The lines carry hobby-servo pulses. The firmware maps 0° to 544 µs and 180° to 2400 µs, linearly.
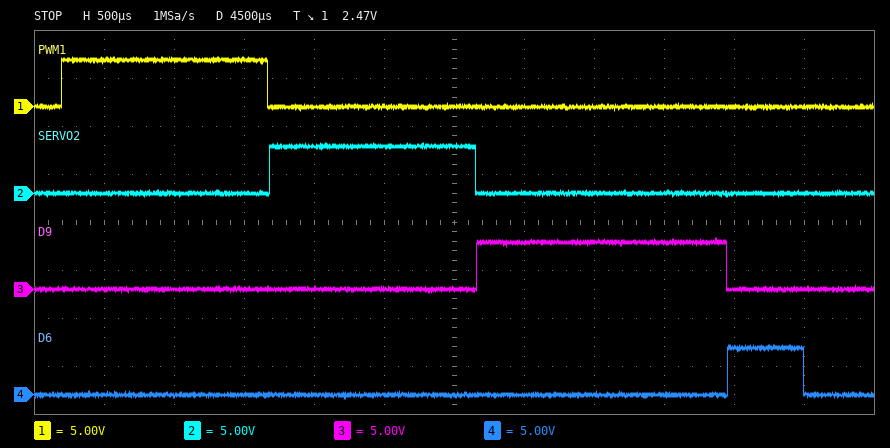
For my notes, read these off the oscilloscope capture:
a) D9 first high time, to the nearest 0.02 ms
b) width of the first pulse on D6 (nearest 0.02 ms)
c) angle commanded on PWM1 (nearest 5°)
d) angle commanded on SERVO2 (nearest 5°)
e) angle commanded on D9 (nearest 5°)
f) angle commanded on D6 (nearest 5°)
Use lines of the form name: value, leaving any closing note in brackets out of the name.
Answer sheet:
D9 first high time, to the nearest 0.02 ms: 1.78 ms
width of the first pulse on D6: 0.54 ms
angle commanded on PWM1: 90°
angle commanded on SERVO2: 90°
angle commanded on D9: 120°
angle commanded on D6: 0°
